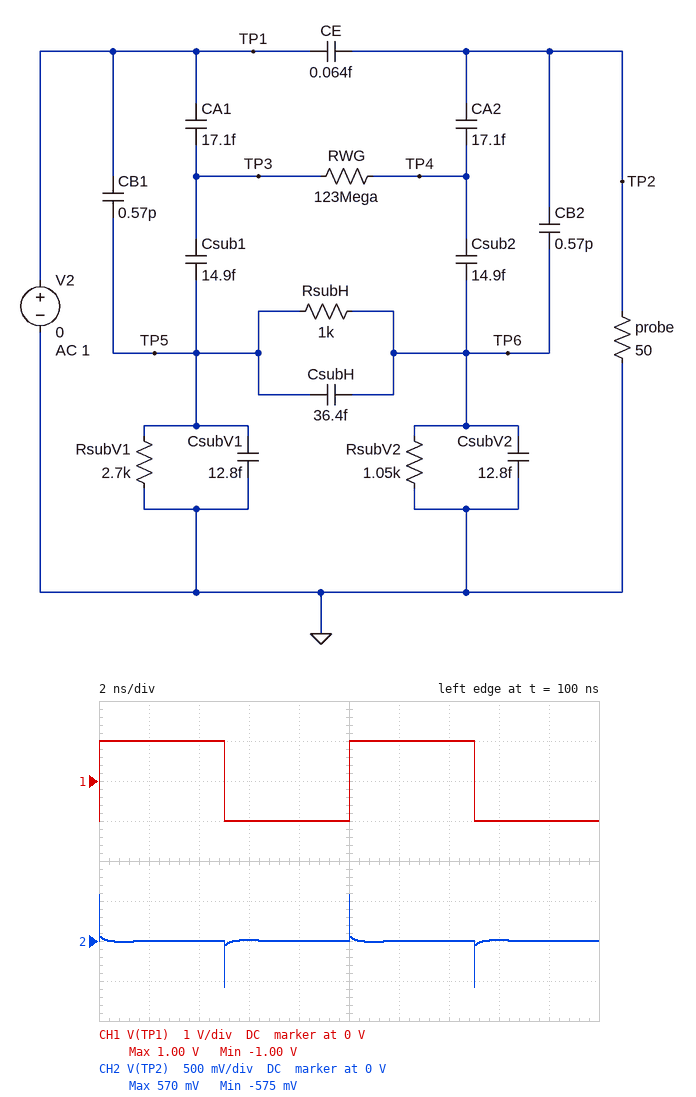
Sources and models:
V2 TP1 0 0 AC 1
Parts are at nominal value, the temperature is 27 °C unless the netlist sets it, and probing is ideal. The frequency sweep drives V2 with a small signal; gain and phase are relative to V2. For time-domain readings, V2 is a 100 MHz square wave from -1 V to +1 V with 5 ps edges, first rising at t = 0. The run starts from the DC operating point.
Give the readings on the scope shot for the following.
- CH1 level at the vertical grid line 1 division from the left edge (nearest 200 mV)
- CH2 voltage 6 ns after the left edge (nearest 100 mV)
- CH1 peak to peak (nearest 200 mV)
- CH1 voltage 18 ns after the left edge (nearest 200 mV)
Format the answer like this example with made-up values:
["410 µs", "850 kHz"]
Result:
["1.0 V", "0 V", "2.0 V", "-1.0 V"]
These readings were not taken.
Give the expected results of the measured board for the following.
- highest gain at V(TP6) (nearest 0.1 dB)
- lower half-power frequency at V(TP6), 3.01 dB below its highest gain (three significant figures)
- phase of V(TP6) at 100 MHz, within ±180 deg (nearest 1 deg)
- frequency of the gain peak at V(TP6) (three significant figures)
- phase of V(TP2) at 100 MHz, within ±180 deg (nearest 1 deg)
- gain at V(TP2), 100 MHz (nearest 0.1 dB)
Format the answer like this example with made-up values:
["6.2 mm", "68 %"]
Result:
["-11.0 dB", "114 MHz", "52 deg", "321 MHz", "141 deg", "-49.6 dB"]
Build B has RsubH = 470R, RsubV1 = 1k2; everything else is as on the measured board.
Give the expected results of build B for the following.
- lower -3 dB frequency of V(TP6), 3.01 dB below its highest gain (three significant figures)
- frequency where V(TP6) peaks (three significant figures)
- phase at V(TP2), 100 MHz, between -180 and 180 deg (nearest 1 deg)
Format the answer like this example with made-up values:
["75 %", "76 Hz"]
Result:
["174 MHz", "525 MHz", "152 deg"]
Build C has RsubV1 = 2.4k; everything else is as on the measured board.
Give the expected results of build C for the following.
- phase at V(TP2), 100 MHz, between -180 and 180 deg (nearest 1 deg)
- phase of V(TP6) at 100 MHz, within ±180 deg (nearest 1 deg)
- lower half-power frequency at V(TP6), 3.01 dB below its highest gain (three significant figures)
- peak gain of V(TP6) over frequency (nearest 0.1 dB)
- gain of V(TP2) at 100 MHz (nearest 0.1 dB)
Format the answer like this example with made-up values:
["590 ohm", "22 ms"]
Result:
["142 deg", "53 deg", "118 MHz", "-11.1 dB", "-49.9 dB"]
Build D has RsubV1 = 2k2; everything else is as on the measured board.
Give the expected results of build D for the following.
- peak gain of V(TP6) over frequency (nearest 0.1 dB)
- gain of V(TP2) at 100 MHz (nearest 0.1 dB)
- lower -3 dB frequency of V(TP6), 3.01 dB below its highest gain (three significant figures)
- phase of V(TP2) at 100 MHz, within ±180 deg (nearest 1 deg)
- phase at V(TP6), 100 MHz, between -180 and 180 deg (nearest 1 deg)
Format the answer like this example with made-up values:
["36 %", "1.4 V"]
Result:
["-11.2 dB", "-50.2 dB", "121 MHz", "143 deg", "54 deg"]
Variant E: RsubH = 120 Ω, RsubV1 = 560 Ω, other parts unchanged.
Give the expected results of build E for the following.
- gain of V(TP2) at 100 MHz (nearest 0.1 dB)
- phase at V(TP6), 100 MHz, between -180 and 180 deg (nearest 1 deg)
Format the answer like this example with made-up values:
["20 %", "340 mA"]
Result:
["-53.3 dB", "74 deg"]
